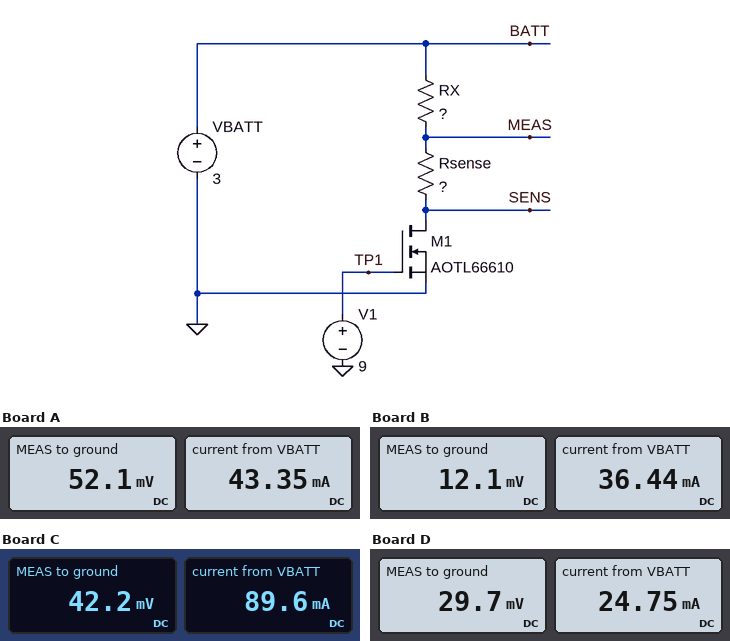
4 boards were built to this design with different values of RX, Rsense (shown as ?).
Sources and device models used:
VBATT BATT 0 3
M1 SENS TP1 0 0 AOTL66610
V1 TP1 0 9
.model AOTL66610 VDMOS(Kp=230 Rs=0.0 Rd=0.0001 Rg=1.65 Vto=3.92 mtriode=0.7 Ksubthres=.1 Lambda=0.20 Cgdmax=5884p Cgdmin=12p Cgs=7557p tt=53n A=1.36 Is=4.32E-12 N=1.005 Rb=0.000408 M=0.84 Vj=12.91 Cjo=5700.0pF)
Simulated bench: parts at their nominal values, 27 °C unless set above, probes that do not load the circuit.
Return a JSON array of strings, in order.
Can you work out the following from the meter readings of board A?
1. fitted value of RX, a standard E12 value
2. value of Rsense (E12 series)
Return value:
["68 Ω", "1.2 Ω"]
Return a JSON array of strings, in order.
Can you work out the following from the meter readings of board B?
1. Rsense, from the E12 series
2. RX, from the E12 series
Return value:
["0.33 Ω", "82 Ω"]
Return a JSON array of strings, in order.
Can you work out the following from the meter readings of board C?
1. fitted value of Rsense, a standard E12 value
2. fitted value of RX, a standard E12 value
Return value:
["0.47 Ω", "33 Ω"]
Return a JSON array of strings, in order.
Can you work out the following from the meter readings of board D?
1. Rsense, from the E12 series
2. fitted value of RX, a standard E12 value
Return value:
["1.2 Ω", "120 Ω"]
